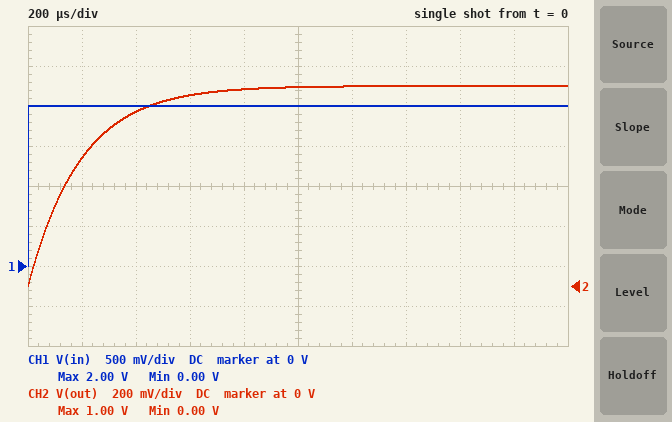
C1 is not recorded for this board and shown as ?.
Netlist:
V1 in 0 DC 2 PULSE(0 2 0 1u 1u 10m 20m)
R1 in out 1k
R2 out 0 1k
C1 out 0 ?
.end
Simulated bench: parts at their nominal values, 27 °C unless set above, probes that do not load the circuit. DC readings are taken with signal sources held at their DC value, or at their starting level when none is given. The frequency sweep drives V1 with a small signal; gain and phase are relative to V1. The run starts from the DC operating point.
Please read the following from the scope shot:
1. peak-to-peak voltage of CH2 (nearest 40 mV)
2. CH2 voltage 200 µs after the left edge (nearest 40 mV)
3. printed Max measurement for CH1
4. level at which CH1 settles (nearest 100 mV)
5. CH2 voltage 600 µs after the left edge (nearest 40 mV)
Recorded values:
1.00 V
640 mV
2.00 V
2.0 V
960 mV
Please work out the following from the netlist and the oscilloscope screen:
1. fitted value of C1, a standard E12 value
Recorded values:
390 nF
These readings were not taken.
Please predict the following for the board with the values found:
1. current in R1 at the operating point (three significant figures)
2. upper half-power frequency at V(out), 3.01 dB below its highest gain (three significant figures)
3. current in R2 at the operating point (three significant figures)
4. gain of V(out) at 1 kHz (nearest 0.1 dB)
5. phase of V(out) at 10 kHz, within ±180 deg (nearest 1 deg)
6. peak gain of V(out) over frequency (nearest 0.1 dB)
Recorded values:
1.00 mA
816 Hz
1.00 mA
-10.0 dB
-85 deg
-6.0 dB
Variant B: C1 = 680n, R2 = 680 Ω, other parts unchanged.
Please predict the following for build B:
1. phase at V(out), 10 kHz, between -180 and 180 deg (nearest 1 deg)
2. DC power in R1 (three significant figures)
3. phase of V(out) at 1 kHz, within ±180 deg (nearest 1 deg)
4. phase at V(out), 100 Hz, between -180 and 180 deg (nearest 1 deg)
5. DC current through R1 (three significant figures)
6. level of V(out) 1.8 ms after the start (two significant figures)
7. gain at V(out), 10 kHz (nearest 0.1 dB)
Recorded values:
-87 deg
1.42 mW
-60 deg
-10 deg
1.19 mA
810 mV
-32.6 dB
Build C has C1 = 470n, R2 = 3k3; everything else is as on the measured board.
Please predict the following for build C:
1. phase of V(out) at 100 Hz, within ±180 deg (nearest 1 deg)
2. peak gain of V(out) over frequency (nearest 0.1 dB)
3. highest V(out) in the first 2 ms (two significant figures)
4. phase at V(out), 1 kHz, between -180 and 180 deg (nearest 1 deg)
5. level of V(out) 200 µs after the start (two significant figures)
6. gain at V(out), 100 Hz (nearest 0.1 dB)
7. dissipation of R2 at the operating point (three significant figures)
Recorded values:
-13 deg
-2.3 dB
1.5 V
-66 deg
650 mV
-2.5 dB
714 µW
